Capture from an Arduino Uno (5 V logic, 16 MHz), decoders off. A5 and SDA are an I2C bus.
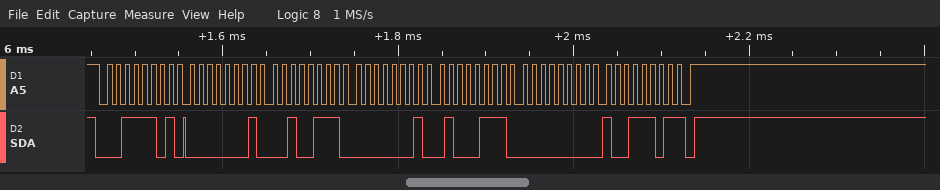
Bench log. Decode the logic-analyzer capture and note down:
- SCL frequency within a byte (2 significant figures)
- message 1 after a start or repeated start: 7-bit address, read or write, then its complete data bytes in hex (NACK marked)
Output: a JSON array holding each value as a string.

["100 kHz", "0x1E read: 01 27 01 47 00 9D NACK"]
